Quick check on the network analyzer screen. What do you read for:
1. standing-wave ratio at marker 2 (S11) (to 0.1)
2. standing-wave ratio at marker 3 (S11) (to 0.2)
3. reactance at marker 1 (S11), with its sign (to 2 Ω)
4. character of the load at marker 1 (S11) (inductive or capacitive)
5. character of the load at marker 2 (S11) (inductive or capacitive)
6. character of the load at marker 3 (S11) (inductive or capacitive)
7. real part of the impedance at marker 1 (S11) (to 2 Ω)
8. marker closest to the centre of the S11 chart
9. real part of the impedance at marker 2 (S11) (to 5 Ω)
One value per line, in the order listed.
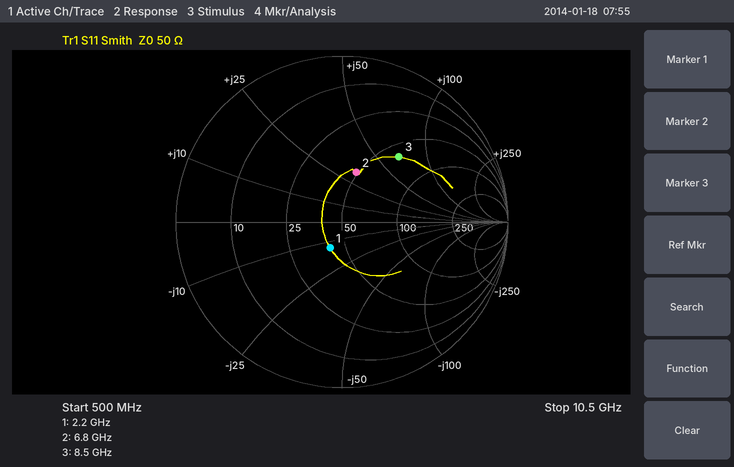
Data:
1.9
3.2
-14 Ω
capacitive
inductive
inductive
42 Ω
marker 1
50 Ω
